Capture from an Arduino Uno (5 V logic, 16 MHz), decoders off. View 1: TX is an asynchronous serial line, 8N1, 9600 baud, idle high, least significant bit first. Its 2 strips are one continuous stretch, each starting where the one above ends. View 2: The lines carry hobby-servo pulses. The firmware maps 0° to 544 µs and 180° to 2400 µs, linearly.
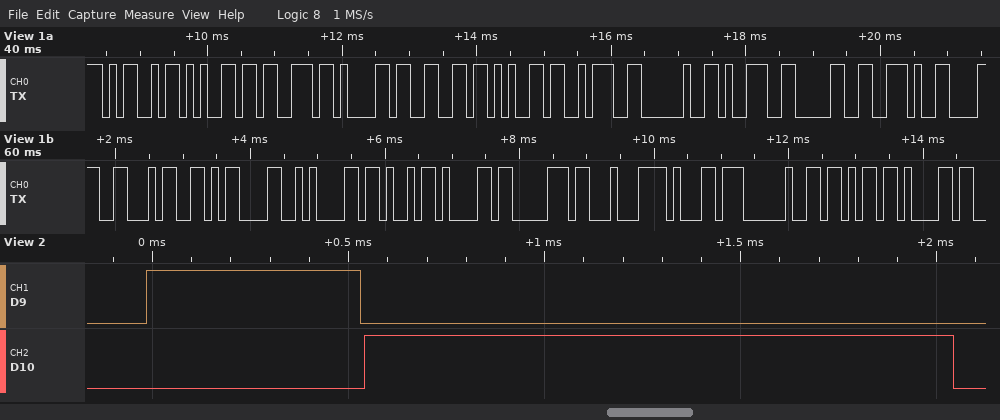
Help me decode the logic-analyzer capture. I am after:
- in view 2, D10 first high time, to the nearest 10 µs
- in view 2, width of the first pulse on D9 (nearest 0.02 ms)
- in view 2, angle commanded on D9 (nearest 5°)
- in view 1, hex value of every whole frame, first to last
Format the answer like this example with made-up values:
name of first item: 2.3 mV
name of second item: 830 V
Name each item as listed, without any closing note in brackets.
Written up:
in view 2, D10 first high time, to the nearest 10 µs: 1500 µs
in view 2, width of the first pulse on D9: 0.54 ms
in view 2, angle commanded on D9: 0°
in view 1, hex value of every whole frame, first to last: 4D 65 73 61 66 65 3A 20 39 30 2E 38 34 0D 0A 4B 61 70 C4 B1 20 6B 61
